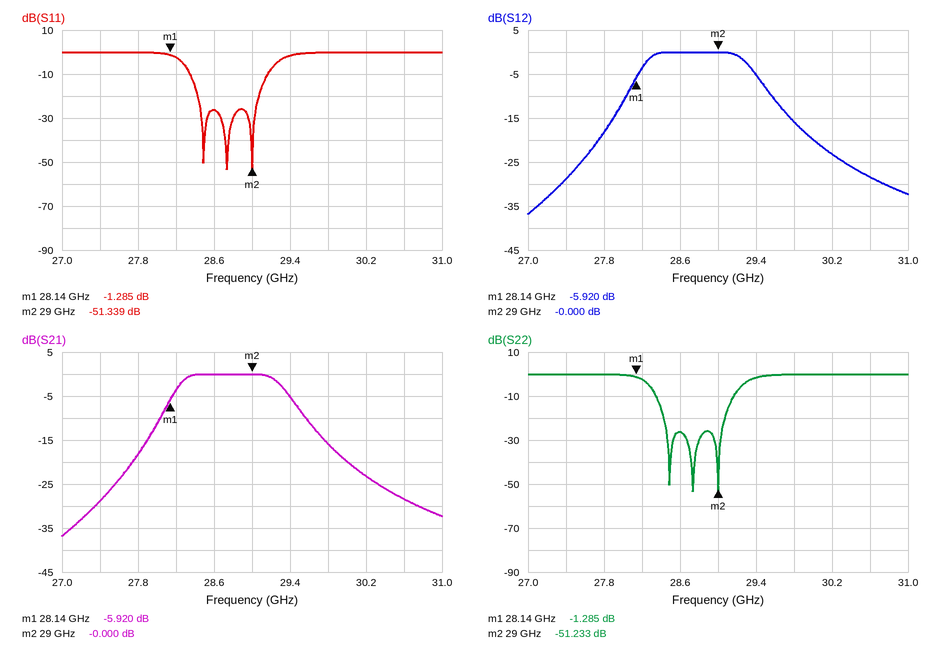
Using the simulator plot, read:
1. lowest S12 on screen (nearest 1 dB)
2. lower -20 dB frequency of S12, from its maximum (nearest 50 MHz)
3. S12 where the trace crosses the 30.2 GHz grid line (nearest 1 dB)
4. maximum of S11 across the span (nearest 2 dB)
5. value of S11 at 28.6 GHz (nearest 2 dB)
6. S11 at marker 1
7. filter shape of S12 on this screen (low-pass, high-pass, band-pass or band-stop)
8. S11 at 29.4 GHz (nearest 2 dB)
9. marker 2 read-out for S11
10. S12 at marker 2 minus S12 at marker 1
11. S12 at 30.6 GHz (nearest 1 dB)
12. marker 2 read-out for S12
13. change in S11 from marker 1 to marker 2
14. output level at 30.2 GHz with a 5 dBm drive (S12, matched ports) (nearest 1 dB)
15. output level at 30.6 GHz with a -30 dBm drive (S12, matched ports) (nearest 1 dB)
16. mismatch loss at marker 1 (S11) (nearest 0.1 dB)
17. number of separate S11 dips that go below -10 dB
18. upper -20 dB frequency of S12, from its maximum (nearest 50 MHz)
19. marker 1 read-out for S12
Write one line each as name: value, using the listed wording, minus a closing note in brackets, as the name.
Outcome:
lowest S12 on screen: -37 dB
lower -20 dB frequency of S12, from its maximum: 27.75 GHz
S12 where the trace crosses the 30.2 GHz grid line: -23 dB
maximum of S11 across the span: 0 dB
value of S11 at 28.6 GHz: -26 dB
S11 at marker 1: -1.285 dB
filter shape of S12 on this screen: band-pass
S11 at 29.4 GHz: -2 dB
marker 2 read-out for S11: -51.339 dB
S12 at marker 2 minus S12 at marker 1: 5.920 dB
S12 at 30.6 GHz: -28 dB
marker 2 read-out for S12: -0.000 dB
change in S11 from marker 1 to marker 2: -50.054 dB
output level at 30.2 GHz with a 5 dBm drive (S12, matched ports): -18 dBm
output level at 30.6 GHz with a -30 dBm drive (S12, matched ports): -58 dBm
mismatch loss at marker 1 (S11): 5.9 dB
number of separate S11 dips that go below -10 dB: 3
upper -20 dB frequency of S12, from its maximum: 30.00 GHz
marker 1 read-out for S12: -5.920 dB
